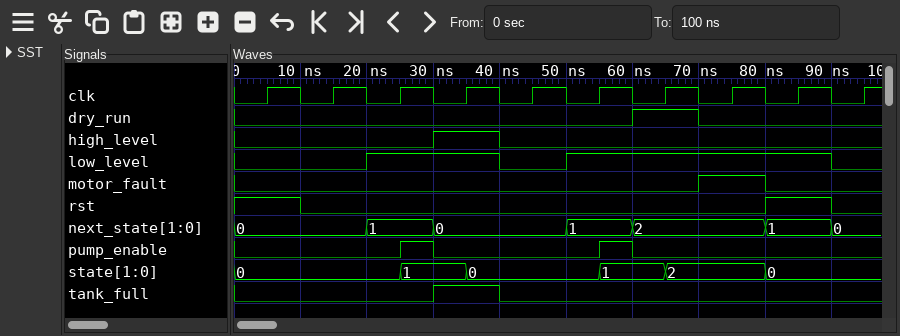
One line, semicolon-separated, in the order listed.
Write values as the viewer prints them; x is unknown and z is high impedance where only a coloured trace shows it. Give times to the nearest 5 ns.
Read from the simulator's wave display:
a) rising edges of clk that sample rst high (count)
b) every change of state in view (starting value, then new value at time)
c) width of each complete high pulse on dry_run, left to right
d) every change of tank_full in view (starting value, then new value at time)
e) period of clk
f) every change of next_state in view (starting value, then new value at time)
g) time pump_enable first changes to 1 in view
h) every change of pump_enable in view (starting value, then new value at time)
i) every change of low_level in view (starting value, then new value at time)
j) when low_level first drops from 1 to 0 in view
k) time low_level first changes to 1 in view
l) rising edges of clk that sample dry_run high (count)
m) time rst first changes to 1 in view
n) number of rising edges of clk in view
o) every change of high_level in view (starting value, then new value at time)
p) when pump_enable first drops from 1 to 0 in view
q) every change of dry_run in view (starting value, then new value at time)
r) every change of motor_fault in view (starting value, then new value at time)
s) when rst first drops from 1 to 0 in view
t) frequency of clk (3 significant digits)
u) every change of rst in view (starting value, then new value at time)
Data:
2; 0, 1 at 25 ns, 0 at 35 ns, 1 at 55 ns, 2 at 65 ns, 0 at 80 ns; 10 ns; 0, 1 at 30 ns, 0 at 40 ns; 10 ns; 0, 1 at 20 ns, 0 at 30 ns, 1 at 50 ns, 2 at 60 ns, 1 at 80 ns, 0 at 90 ns; 25 ns; 0, 1 at 25 ns, 0 at 30 ns, 1 at 55 ns, 0 at 60 ns; 0, 1 at 20 ns, 0 at 40 ns, 1 at 50 ns, 0 at 90 ns; 40 ns; 20 ns; 1; 80 ns; 10; 0, 1 at 30 ns, 0 at 40 ns; 30 ns; 0, 1 at 60 ns, 0 at 70 ns; 0, 1 at 70 ns, 0 at 80 ns; 10 ns; 100 MHz; 1, 0 at 10 ns, 1 at 80 ns, 0 at 90 ns
